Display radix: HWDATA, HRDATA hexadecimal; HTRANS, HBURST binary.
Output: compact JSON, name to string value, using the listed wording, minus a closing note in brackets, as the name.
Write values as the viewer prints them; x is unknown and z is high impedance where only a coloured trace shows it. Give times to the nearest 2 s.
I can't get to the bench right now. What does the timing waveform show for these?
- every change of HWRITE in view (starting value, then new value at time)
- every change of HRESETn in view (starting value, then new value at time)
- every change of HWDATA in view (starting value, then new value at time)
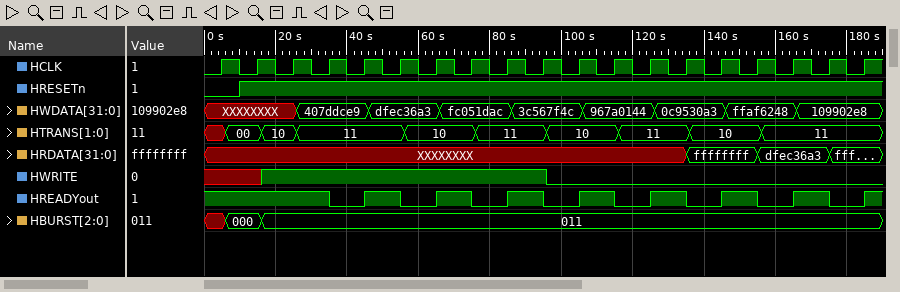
{"every change of HWRITE in view": "x, 1 at 16 s, 0 at 96 s", "every change of HRESETn in view": "0, 1 at 10 s", "every change of HWDATA in view": "XXXXXXXX, 407ddce9 at 26 s, dfec36a3 at 46 s, fc051dac at 66 s, 3c567f4c at 86 s, 967a0144 at 106 s, 0c9530a3 at 126 s, ffaf6248 at 146 s, 109902e8 at 166 s"}
